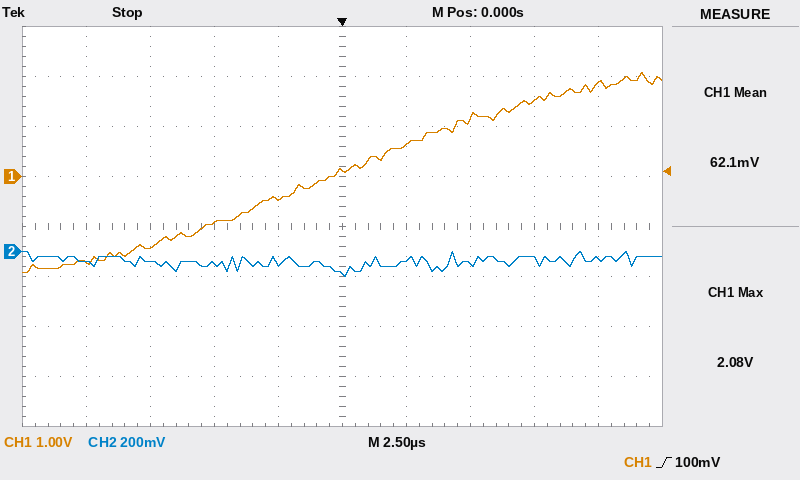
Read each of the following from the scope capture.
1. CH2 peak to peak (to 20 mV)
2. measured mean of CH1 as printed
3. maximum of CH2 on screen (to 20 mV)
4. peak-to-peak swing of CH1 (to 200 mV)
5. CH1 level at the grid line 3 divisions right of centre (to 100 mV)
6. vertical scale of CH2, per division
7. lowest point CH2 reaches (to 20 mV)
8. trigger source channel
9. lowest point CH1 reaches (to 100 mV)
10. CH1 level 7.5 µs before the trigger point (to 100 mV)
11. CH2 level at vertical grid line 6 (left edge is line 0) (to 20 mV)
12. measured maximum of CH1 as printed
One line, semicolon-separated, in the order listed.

100 mV; 62.1 mV; 0 mV; 4.0 V; 1.5 V; 200 mV; -100 mV; CH1; -1.9 V; -1.4 V; -40 mV; 2.08 V
